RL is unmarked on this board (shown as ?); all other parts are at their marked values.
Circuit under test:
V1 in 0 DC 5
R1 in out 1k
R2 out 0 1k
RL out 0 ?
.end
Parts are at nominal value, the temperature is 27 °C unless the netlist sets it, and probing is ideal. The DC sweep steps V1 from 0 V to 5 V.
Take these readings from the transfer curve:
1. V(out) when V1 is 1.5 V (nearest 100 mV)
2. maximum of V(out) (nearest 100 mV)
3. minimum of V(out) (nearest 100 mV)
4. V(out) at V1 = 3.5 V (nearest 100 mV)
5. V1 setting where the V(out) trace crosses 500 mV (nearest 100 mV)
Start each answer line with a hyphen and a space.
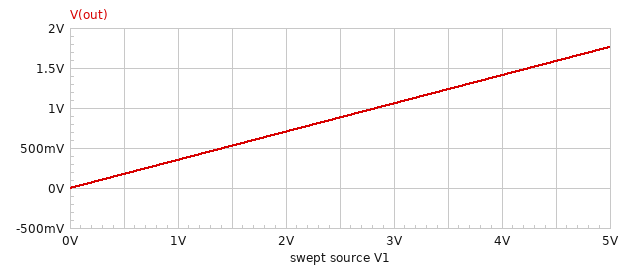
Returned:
- 500 mV
- 1.8 V
- 0 V
- 1.2 V
- 1.4 V
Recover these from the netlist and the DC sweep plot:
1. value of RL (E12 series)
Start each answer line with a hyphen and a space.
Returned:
- 1.2 kΩ
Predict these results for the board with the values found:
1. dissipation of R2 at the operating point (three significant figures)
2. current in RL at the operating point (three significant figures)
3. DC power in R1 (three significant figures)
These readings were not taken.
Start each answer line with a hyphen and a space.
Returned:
- 3.11 mW
- 1.47 mA
- 10.5 mW
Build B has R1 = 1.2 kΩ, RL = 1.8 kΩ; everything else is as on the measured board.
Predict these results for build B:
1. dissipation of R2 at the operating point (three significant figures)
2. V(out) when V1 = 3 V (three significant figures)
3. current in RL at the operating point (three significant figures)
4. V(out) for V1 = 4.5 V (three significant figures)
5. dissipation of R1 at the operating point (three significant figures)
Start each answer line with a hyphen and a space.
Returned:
- 3.04 mW
- 1.05 V
- 969 µA
- 1.57 V
- 8.83 mW
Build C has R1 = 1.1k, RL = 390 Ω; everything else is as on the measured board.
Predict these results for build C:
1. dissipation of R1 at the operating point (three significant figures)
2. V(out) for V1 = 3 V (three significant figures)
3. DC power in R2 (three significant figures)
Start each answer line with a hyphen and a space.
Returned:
- 14.4 mW
- 610 mV
- 1.03 mW
